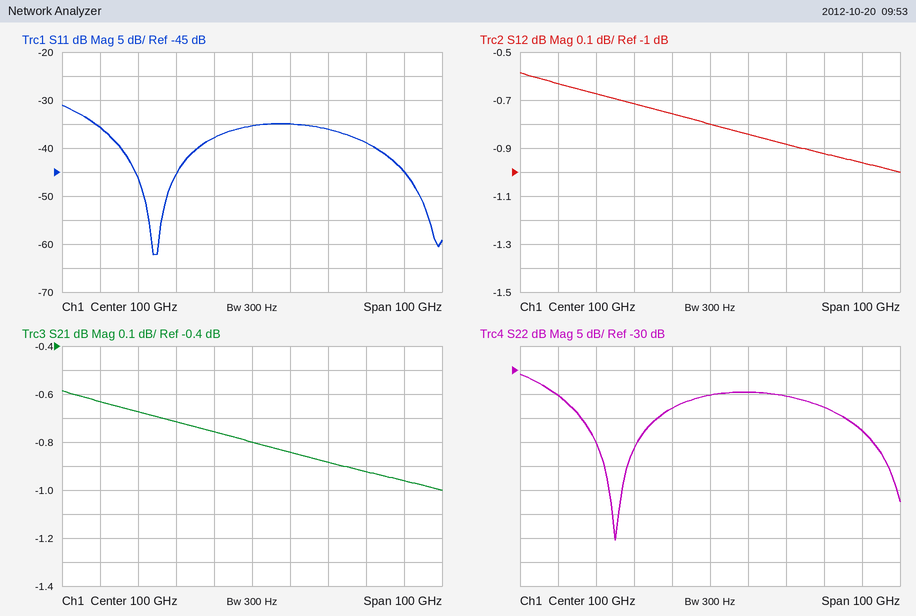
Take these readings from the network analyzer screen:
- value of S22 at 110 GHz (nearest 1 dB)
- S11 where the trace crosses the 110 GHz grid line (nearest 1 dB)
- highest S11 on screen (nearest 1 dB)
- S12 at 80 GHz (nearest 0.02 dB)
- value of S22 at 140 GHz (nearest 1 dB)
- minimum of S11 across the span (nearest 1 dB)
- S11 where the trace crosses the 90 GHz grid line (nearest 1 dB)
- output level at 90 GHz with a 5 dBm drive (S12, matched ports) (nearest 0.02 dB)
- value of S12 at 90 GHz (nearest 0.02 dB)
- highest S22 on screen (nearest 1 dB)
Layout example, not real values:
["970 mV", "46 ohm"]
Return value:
["-35 dB", "-35 dB", "-31 dB", "-0.72 dB", "-43 dB", "-62 dB", "-38 dB", "4.24 dBm", "-0.76 dB", "-31 dB"]
